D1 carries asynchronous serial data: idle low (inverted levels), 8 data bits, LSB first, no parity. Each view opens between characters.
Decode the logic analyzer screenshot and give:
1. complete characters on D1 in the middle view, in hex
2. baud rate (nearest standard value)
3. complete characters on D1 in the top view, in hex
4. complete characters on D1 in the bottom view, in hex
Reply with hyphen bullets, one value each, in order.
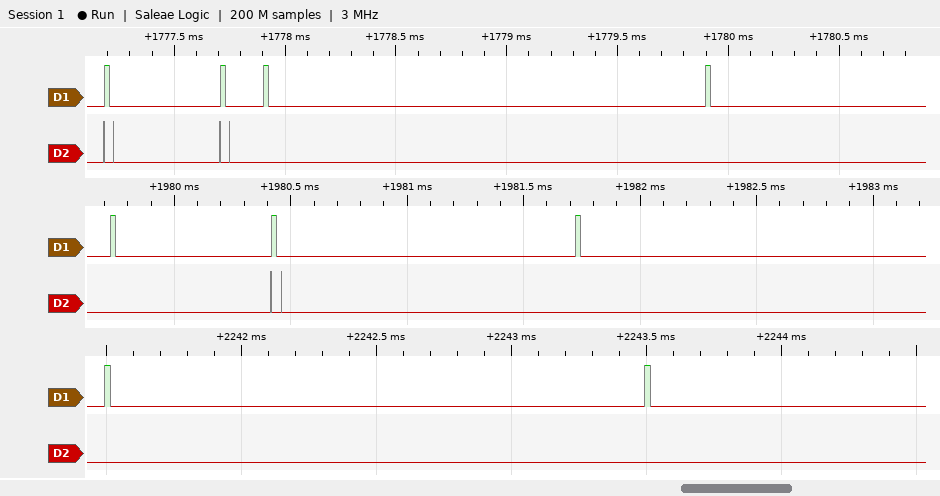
- FF, FF, FF
- 38400 baud
- FF, BF, FF
- FF, FF
